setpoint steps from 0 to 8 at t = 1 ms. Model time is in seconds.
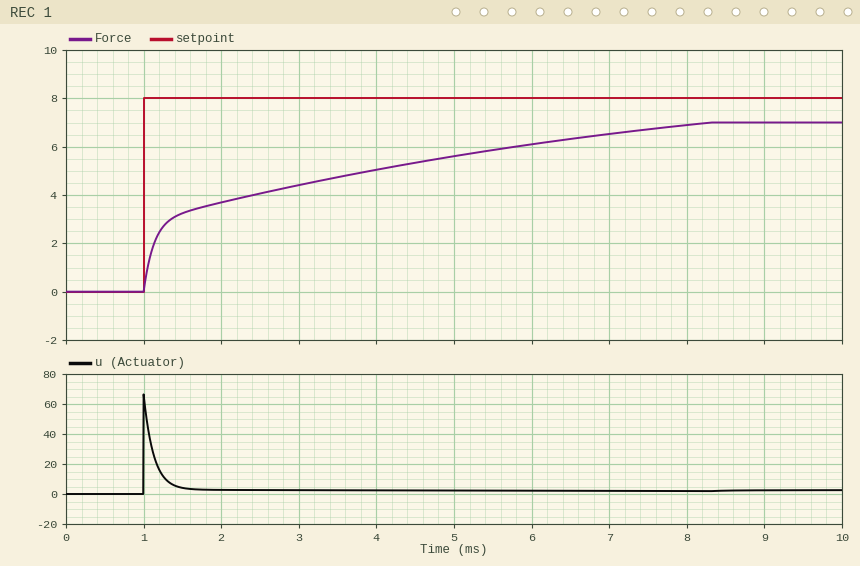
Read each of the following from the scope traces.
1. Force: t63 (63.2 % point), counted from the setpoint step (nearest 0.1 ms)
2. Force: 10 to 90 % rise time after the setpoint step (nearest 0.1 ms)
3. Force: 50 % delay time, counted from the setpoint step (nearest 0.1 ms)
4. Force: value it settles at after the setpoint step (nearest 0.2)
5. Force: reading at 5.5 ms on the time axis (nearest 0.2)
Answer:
2.0 ms
5.4 ms
0.8 ms
7.0
5.8
